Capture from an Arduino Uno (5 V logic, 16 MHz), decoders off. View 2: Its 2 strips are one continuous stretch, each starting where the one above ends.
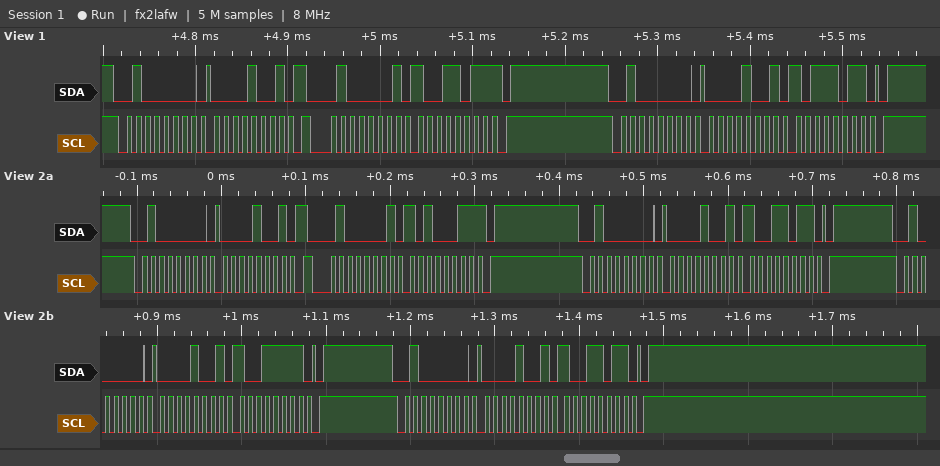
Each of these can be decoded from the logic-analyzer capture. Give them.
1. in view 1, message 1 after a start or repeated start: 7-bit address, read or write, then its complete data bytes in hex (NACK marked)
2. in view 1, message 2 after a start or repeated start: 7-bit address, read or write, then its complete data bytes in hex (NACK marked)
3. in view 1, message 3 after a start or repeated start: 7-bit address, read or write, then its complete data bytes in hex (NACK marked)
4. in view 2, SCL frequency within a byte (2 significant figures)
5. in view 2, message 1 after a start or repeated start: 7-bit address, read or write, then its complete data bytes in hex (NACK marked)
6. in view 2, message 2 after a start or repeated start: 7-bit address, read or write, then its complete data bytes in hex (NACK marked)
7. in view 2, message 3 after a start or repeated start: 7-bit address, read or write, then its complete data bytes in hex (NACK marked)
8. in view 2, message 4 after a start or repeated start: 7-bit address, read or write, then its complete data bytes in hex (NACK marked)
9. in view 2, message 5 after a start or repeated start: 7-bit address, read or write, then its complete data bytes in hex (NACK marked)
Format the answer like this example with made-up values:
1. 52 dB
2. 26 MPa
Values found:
1. 0x20 write: 09
2. 0x20 read: 9B NACK
3. 0x20 write: 09 BB
4. 100 kHz
5. 0x20 write: 09
6. 0x20 read: A3 NACK
7. 0x20 write: 09 9B
8. 0x20 write: 09 9F
9. 0x20 write: 09 9B
